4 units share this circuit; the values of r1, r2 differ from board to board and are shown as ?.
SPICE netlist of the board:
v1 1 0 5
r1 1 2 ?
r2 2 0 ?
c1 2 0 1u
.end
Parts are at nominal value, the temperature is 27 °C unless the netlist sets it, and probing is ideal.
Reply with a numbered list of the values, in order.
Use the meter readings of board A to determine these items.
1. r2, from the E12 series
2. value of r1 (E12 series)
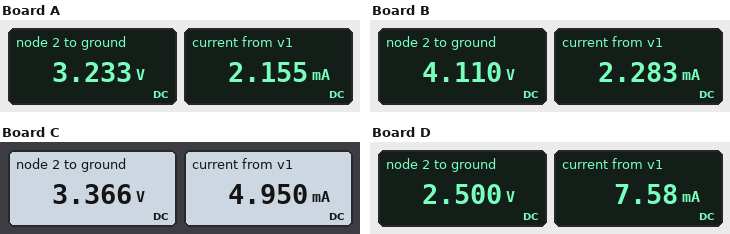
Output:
1. 1.5 kΩ
2. 820 Ω
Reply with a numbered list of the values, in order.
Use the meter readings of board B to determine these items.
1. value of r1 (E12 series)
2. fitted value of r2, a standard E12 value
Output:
1. 390 Ω
2. 1.8 kΩ
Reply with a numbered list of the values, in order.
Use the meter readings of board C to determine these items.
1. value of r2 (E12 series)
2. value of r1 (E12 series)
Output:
1. 680 Ω
2. 330 Ω
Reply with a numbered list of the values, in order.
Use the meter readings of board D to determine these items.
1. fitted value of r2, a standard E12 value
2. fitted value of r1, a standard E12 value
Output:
1. 330 Ω
2. 330 Ω
